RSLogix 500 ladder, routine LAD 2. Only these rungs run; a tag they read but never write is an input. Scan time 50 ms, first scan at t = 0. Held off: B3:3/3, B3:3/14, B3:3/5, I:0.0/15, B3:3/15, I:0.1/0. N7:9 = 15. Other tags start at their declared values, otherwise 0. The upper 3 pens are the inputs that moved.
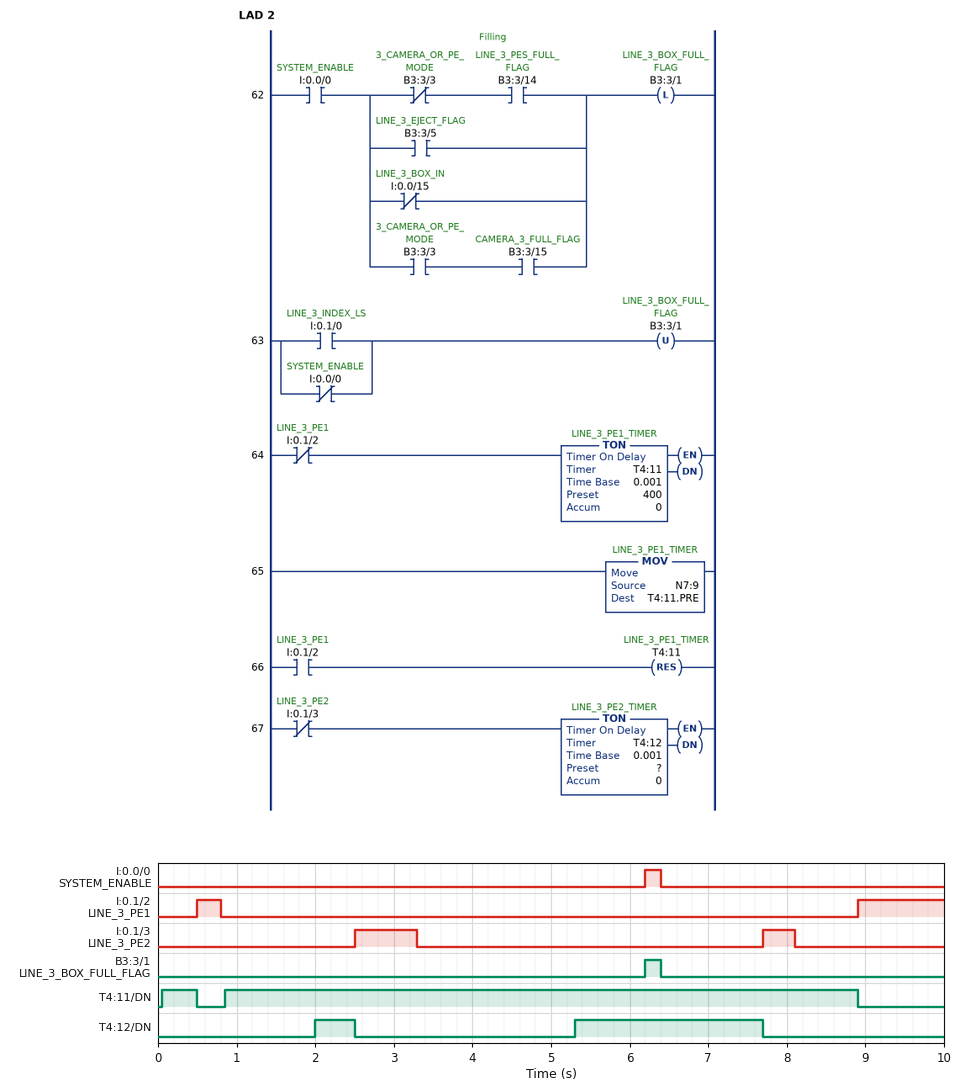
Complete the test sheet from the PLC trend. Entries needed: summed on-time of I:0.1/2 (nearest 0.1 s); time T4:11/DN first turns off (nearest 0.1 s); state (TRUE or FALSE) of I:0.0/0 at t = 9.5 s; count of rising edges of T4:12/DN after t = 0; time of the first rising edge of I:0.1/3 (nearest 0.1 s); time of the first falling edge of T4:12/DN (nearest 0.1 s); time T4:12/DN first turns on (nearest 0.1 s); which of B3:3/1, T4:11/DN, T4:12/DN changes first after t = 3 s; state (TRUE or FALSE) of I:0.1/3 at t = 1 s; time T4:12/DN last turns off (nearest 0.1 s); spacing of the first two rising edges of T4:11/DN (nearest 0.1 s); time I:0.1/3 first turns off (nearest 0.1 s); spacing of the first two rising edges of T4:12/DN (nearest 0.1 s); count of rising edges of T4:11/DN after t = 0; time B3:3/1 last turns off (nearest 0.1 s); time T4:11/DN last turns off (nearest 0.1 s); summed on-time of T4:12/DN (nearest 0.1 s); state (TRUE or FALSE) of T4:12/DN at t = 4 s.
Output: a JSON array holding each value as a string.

["1.4 s", "0.5 s", "FALSE", "2", "2.5 s", "2.5 s", "2.0 s", "T4:12/DN", "FALSE", "7.7 s", "0.8 s", "3.3 s", "3.3 s", "2", "6.4 s", "8.9 s", "2.9 s", "FALSE"]
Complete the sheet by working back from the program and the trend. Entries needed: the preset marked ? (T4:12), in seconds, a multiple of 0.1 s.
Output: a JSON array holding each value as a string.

["2.0 s"]
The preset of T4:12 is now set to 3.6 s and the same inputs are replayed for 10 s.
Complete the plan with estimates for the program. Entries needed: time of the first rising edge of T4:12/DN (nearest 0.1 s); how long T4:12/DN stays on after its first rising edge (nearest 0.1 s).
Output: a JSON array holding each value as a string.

["6.9 s", "0.8 s"]
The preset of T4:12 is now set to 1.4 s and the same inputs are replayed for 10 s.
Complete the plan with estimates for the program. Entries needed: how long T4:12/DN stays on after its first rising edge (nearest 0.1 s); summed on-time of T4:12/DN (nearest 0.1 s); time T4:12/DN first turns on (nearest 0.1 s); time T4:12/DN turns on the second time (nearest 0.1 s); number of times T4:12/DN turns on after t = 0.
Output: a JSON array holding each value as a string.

["1.1 s", "4.6 s", "1.4 s", "4.7 s", "3"]
